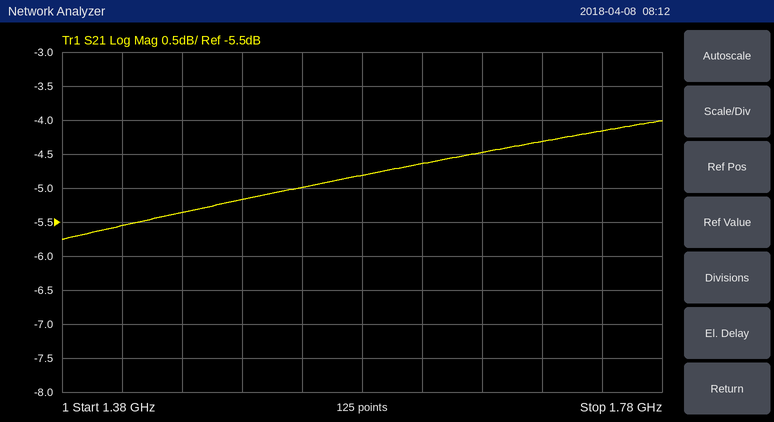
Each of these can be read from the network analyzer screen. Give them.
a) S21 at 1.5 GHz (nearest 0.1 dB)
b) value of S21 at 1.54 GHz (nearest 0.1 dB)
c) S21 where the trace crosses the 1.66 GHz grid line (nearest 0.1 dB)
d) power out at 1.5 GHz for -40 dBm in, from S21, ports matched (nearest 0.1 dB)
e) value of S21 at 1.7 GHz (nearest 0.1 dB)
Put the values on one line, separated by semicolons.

-5.2 dB; -5.0 dB; -4.5 dB; -45.2 dBm; -4.3 dB
